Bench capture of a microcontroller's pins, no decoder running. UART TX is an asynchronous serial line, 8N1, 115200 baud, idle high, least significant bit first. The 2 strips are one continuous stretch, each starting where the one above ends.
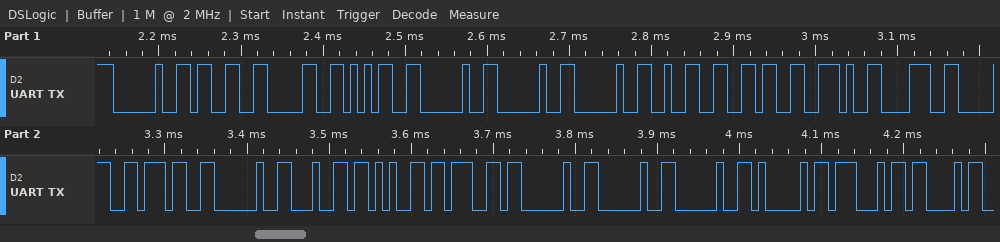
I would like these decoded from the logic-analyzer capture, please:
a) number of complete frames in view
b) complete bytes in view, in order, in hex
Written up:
23
20 33 30 35 20 20 20 32 36 2E 38 30 37 20 64 65 67 20 20 20 41 47 43
